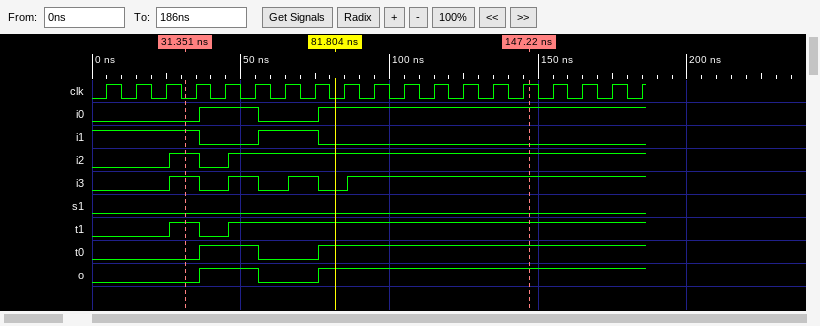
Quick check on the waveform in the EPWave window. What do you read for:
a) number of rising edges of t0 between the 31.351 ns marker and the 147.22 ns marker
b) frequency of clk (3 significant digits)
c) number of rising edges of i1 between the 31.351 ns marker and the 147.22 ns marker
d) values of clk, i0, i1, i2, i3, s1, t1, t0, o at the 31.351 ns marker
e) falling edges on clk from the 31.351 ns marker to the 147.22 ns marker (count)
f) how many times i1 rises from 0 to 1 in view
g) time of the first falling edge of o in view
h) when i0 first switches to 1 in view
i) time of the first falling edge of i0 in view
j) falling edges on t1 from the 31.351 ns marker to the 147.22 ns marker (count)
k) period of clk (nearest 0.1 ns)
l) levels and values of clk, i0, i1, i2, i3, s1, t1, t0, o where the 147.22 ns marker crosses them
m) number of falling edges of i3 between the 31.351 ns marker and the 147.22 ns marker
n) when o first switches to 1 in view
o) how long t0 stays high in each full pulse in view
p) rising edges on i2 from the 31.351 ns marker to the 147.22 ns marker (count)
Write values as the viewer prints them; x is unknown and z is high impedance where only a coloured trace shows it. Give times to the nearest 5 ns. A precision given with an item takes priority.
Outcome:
2
100 MHz
1
clk=0, i0=0, i1=1, i2=1, i3=1, s1=0, t1=1, t0=0, o=0
11
1
55 ns
35 ns
55 ns
1
10 ns
clk=1, i0=1, i1=0, i2=1, i3=1, s1=0, t1=1, t0=1, o=1
3
35 ns
20 ns
1
